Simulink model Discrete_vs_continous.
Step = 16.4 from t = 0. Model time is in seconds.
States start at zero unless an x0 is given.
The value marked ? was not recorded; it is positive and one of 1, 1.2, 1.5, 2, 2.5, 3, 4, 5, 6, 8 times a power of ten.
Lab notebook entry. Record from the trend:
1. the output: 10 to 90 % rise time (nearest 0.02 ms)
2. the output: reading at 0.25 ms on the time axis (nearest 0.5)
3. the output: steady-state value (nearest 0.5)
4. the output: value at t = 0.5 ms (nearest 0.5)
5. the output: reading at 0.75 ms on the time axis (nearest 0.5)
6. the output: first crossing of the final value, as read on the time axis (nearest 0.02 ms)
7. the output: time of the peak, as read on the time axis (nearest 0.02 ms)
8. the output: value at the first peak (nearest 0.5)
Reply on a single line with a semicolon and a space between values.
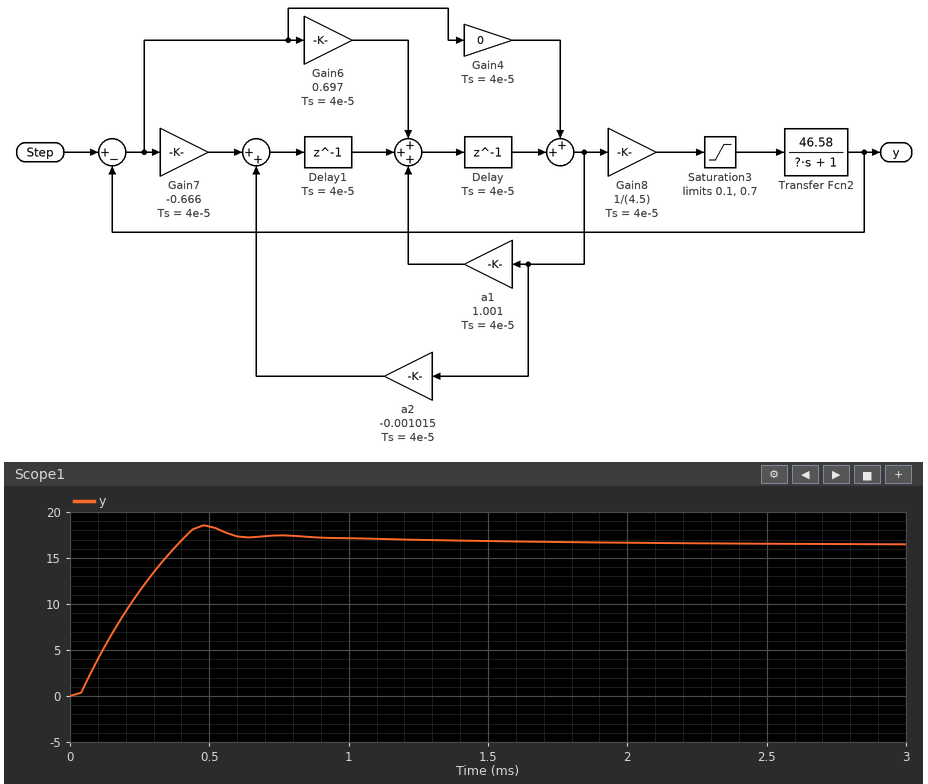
0.28 ms; 11.5; 16.5; 18.5; 17.5; 0.38 ms; 0.48 ms; 18.5
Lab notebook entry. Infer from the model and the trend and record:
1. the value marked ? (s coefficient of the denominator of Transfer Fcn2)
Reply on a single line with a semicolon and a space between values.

0.0005
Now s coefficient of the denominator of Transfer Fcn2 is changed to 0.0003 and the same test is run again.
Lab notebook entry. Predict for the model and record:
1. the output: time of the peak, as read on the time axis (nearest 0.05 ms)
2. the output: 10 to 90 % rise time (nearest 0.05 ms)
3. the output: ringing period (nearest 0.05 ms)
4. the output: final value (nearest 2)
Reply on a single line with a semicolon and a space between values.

0.30 ms; 0.15 ms; 0.25 ms; 16
